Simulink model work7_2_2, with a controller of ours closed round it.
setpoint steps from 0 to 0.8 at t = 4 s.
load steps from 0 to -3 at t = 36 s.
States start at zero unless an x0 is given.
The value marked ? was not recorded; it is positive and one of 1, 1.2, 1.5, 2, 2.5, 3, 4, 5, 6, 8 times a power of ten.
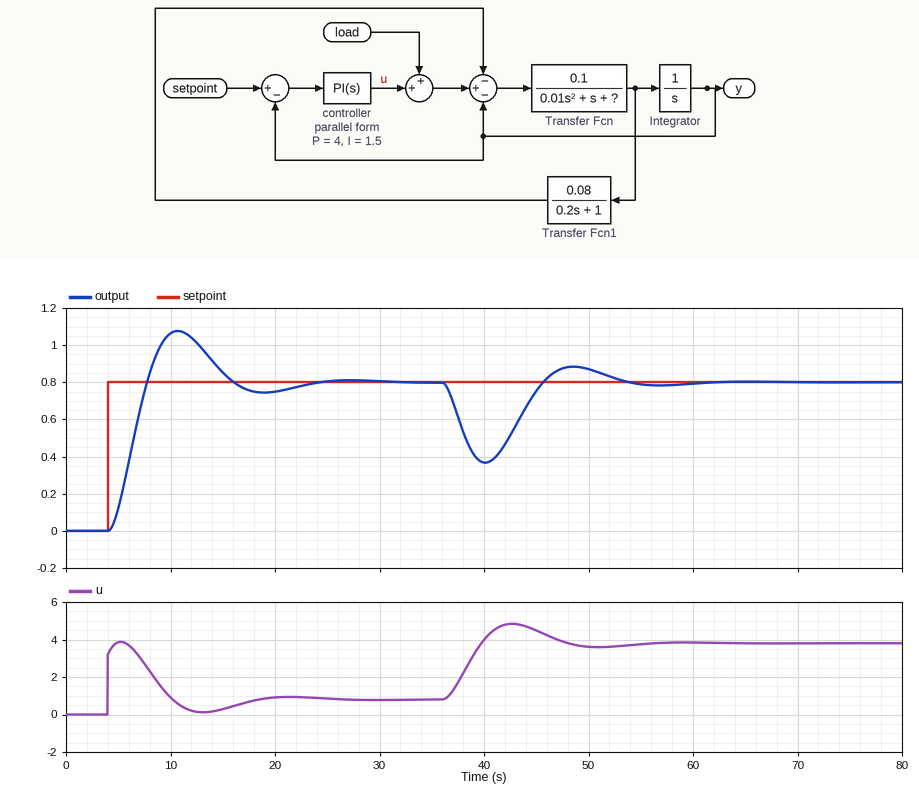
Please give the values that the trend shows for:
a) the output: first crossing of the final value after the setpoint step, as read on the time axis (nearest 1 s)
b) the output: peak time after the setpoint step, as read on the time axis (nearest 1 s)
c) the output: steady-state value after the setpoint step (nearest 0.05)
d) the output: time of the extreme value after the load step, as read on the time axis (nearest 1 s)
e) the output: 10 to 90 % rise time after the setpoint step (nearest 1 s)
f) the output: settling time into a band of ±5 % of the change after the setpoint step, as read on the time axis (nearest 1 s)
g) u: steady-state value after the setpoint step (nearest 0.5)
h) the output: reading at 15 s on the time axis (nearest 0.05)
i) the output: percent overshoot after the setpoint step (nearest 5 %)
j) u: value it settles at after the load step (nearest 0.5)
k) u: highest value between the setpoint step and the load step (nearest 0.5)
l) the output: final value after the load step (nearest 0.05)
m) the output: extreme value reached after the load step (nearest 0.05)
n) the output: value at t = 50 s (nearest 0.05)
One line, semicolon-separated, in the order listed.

8 s; 11 s; 0.80; 40 s; 3 s; 21 s; 1.0; 0.85; 35 %; 4.0; 4.0; 0.80; 0.35; 0.85
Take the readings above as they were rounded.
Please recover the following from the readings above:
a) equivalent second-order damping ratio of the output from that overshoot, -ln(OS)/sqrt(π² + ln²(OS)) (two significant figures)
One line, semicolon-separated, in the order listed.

0.32
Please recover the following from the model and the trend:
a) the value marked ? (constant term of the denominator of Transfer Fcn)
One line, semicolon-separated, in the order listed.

1.2
